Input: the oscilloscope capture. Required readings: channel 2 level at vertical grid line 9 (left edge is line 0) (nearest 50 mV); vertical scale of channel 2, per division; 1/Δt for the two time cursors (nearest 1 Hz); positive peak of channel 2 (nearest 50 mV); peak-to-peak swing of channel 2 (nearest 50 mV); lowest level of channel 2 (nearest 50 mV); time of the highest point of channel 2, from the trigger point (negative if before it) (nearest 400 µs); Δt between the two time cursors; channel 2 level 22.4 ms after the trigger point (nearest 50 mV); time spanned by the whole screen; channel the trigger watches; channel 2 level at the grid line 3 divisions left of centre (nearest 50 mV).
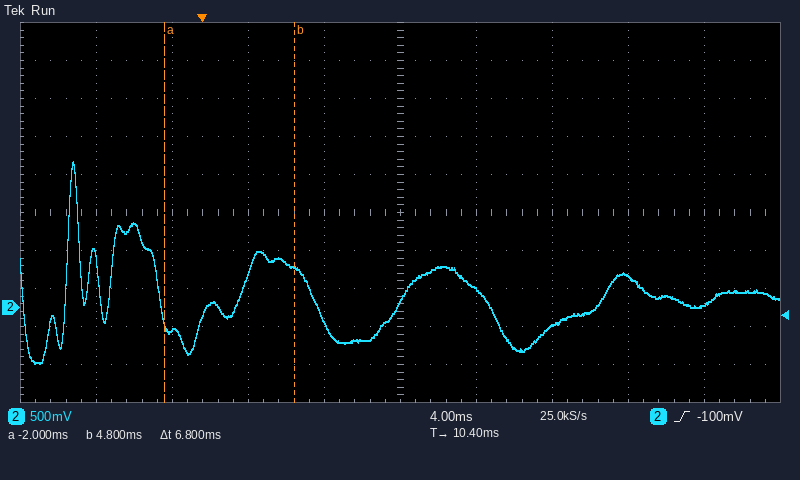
50 mV
500 mV
147 Hz
1.90 V
2.65 V
-750 mV
-6.8 ms
6.8 ms
400 mV
40 ms
channel 2
-300 mV
